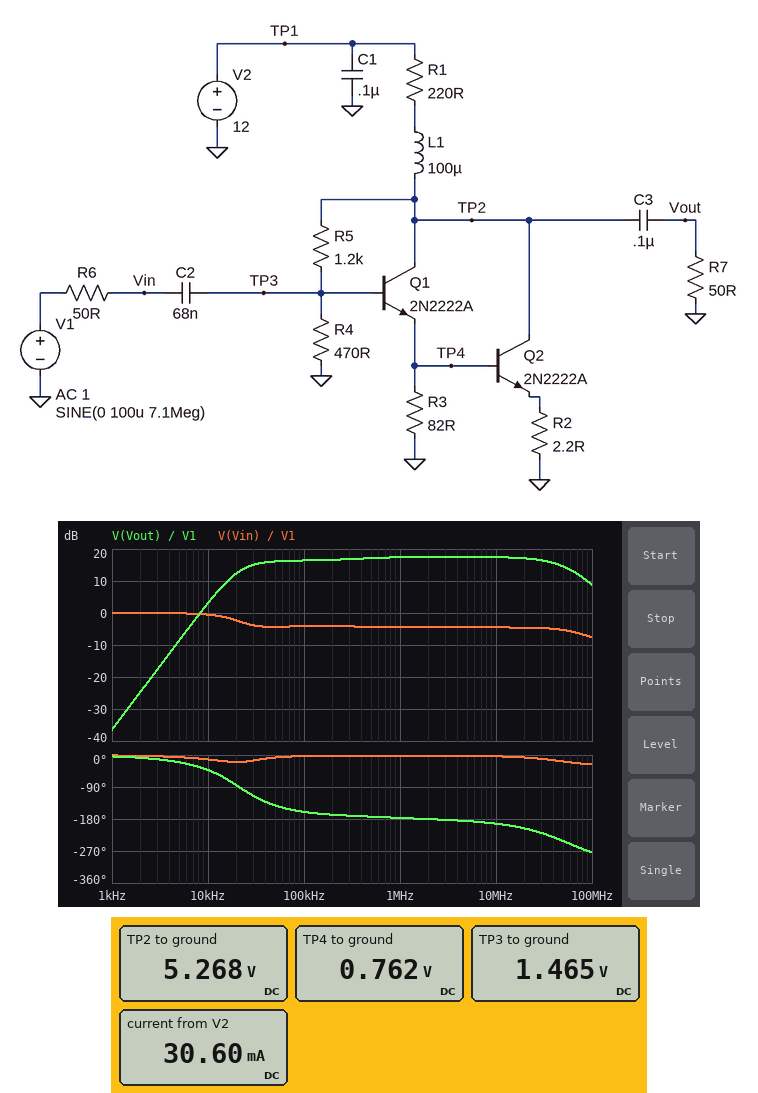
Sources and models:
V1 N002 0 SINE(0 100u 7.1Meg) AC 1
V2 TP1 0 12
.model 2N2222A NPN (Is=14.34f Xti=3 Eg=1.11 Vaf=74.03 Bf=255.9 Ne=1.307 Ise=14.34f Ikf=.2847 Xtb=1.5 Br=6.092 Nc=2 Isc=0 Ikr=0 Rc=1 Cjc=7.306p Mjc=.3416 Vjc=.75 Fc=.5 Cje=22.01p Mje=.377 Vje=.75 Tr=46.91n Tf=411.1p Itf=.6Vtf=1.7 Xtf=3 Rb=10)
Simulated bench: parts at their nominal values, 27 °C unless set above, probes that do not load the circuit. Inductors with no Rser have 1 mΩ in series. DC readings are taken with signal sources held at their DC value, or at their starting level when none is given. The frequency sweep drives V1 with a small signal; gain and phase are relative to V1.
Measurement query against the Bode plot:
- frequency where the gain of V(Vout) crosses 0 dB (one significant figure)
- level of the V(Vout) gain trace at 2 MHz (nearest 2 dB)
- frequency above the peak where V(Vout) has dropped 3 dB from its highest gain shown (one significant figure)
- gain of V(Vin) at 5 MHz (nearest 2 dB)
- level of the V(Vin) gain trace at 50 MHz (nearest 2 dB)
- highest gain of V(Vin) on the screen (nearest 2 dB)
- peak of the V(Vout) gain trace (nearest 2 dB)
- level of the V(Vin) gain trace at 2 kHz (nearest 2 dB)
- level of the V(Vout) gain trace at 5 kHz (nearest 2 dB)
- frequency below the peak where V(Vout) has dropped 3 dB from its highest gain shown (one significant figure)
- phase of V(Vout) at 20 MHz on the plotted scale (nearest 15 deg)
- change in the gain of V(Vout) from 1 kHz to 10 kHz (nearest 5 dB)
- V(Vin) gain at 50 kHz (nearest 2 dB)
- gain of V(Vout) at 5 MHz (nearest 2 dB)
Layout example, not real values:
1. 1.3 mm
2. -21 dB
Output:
1. 8 kHz
2. 18 dB
3. 50 MHz
4. -4 dB
5. -6 dB
6. 0 dB
7. 18 dB
8. 0 dB
9. -8 dB
10. 30 kHz
11. -210 deg
12. 40 dB
13. -4 dB
14. 18 dB
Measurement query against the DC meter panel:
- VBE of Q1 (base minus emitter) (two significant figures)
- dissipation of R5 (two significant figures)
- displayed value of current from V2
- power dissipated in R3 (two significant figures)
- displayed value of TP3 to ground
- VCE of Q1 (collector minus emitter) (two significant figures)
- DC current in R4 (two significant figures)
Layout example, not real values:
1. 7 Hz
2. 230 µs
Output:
1. 700 mV
2. 12 mW
3. 30.60 mA
4. 7.1 mW
5. 1.465 V
6. 4.5 V
7. 3.1 mA
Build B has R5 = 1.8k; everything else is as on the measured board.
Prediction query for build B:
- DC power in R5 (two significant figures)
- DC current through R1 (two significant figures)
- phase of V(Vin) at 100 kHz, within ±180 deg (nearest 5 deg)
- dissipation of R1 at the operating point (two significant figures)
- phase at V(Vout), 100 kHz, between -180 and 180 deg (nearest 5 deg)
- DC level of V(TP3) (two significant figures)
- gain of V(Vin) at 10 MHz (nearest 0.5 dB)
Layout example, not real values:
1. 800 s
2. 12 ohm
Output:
1. 17 mW
2. 23 mA
3. 0 deg
4. 110 mW
5. -165 deg
6. 1.4 V
7. -3.0 dB
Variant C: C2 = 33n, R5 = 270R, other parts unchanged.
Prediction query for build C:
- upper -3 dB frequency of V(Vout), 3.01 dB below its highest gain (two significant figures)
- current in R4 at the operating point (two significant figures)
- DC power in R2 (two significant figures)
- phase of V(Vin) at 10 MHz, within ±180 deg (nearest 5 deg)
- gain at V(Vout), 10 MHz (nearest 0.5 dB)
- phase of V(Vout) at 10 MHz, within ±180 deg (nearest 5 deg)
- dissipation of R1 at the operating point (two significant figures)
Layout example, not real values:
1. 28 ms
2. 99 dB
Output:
1. 80 MHz
2. 3.2 mA
3. 2.1 mW
4. 5 deg
5. 11.0 dB
6. 170 deg
7. 420 mW
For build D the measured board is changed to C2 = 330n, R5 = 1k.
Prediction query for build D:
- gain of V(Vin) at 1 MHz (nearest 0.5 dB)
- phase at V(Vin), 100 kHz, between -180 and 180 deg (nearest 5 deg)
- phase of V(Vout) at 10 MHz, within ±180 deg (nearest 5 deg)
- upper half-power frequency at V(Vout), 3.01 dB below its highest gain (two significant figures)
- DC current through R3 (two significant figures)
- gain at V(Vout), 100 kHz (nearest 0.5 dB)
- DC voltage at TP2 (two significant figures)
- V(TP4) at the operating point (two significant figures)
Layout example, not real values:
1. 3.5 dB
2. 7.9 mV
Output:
1. -5.0 dB
2. 0 deg
3. 165 deg
4. 51 MHz
5. 9.4 mA
6. 16.0 dB
7. 4.7 V
8. 770 mV
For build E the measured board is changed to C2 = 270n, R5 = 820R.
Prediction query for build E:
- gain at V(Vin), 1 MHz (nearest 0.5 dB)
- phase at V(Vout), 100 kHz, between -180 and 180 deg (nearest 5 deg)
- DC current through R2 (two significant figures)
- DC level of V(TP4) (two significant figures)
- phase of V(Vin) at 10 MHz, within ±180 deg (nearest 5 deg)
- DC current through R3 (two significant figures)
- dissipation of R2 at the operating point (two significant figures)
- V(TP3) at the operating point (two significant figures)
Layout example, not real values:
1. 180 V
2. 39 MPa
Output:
1. -6.0 dB
2. -165 deg
3. 23 mA
4. 780 mV
5. 0 deg
6. 9.5 mA
7. 1.2 mW
8. 1.5 V
